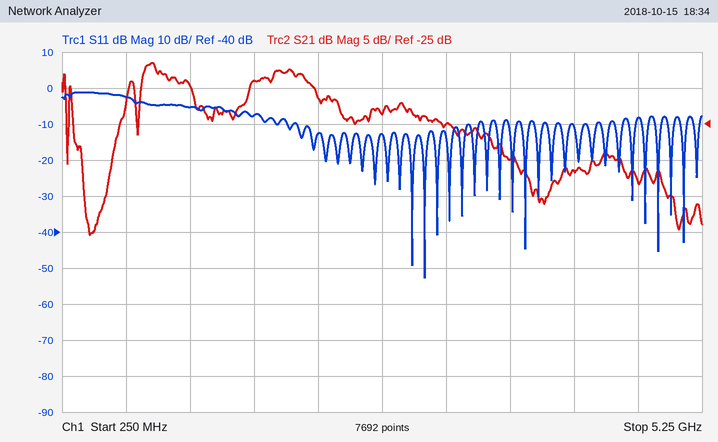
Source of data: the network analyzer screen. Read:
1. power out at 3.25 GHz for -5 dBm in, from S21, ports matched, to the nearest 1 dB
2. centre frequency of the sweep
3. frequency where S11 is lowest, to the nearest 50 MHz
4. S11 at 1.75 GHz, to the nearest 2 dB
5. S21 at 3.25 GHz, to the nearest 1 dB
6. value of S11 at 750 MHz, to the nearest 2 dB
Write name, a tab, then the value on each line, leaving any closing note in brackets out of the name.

power out at 3.25 GHz for -5 dBm in, from S21, ports matched, to the nearest 1 dB	-30 dBm
centre frequency of the sweep	2.75 GHz
frequency where S11 is lowest, to the nearest 50 MHz	3.10 GHz
S11 at 1.75 GHz, to the nearest 2 dB	-8 dB
S21 at 3.25 GHz, to the nearest 1 dB	-25 dB
value of S11 at 750 MHz, to the nearest 2 dB	-2 dB
